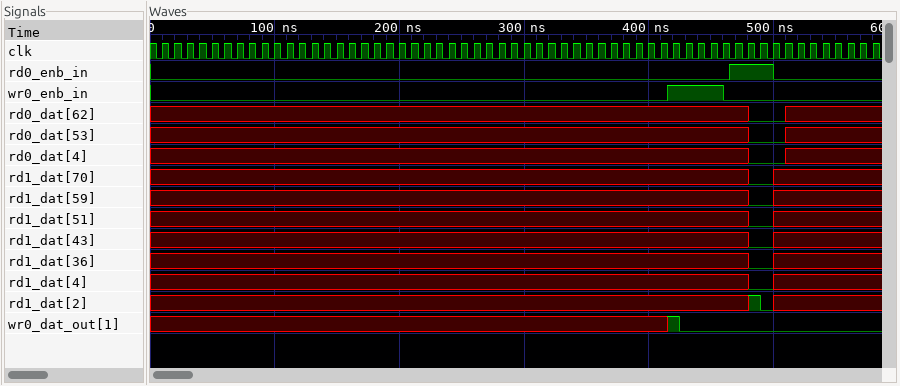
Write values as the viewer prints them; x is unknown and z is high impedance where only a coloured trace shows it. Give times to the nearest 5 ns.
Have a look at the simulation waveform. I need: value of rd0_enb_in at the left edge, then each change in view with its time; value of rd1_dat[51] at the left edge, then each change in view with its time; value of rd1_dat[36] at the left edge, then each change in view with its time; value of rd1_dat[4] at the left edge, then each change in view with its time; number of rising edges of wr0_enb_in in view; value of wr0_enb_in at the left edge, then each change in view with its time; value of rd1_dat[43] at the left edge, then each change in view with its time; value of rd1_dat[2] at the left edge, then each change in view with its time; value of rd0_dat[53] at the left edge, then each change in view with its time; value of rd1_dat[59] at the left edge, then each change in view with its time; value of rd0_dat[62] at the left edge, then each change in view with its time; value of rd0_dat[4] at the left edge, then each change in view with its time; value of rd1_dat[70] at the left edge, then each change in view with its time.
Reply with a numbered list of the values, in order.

1. 0, 1 at 465 ns, 0 at 500 ns
2. x, 0 at 480 ns, x at 500 ns
3. x, 0 at 480 ns, x at 500 ns
4. x, 0 at 480 ns, x at 500 ns
5. 1
6. 0, 1 at 415 ns, 0 at 460 ns
7. x, 0 at 480 ns, x at 500 ns
8. x, 1 at 480 ns, 0 at 490 ns, x at 500 ns
9. x, 0 at 480 ns, x at 510 ns
10. x, 0 at 480 ns, x at 500 ns
11. x, 0 at 480 ns, x at 510 ns
12. x, 0 at 480 ns, x at 510 ns
13. x, 0 at 480 ns, x at 500 ns
